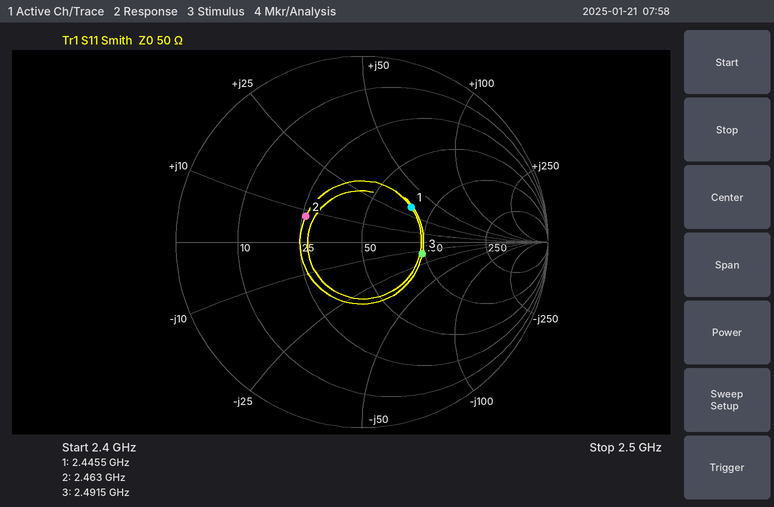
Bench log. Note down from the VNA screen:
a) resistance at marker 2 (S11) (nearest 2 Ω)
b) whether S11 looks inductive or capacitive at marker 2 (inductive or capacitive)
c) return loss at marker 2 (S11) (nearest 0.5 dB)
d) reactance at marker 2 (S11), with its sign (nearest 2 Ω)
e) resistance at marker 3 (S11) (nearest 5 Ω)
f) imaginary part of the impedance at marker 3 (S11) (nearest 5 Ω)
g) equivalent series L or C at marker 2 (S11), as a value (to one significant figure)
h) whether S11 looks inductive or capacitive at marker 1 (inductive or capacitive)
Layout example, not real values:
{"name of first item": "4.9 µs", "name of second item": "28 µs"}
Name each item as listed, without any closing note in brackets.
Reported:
{"resistance at marker 2 (S11)": "26 Ω", "whether S11 looks inductive or capacitive at marker 2": "inductive", "return loss at marker 2 (S11)": "9.5 dB", "reactance at marker 2 (S11), with its sign": "+8 Ω", "resistance at marker 3 (S11)": "95 Ω", "imaginary part of the impedance at marker 3 (S11)": "-15 Ω", "equivalent series L or C at marker 2 (S11), as a value": "500 pH", "whether S11 looks inductive or capacitive at marker 1": "inductive"}
